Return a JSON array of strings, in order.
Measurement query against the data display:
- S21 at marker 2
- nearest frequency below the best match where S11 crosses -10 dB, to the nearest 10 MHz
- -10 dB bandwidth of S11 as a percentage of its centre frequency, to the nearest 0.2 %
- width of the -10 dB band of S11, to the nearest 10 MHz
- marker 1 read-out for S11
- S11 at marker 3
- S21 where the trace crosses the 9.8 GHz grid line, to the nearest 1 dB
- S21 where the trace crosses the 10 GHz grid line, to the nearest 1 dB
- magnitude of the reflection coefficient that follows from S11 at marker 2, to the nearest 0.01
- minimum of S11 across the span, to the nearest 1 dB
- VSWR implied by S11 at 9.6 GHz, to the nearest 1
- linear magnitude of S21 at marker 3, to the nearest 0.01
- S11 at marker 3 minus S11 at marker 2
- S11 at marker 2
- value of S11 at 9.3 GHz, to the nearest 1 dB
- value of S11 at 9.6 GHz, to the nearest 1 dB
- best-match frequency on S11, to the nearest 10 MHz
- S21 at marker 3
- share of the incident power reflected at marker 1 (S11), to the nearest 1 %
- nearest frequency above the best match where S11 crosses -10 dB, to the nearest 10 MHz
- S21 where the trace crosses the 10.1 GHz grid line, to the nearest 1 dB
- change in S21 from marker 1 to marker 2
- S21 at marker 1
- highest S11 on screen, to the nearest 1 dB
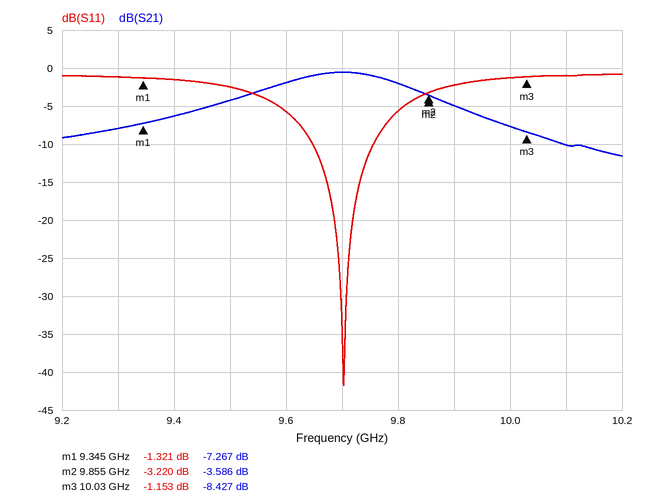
["-3.586 dB", "9.65 GHz", "1.2 %", "110 MHz", "-1.321 dB", "-1.153 dB", "-2 dB", "-8 dB", "0.69", "-42 dB", "3", "0.38", "2.067 dB", "-3.220 dB", "-1 dB", "-6 dB", "9.70 GHz", "-8.427 dB", "74 %", "9.76 GHz", "-10 dB", "3.681 dB", "-7.267 dB", "-1 dB"]
